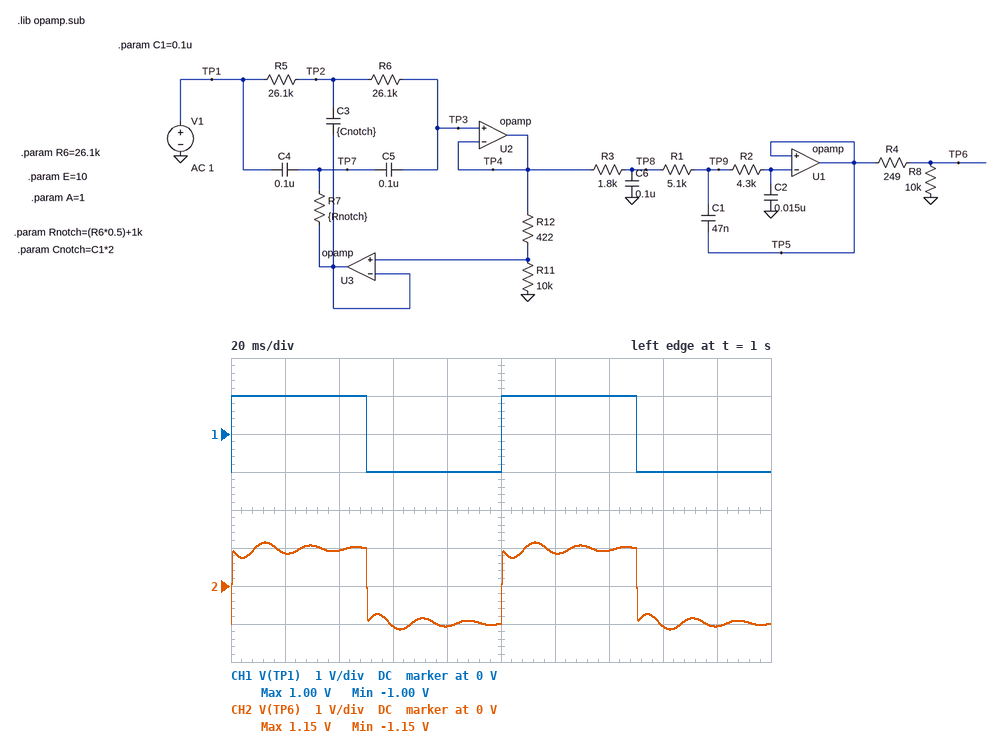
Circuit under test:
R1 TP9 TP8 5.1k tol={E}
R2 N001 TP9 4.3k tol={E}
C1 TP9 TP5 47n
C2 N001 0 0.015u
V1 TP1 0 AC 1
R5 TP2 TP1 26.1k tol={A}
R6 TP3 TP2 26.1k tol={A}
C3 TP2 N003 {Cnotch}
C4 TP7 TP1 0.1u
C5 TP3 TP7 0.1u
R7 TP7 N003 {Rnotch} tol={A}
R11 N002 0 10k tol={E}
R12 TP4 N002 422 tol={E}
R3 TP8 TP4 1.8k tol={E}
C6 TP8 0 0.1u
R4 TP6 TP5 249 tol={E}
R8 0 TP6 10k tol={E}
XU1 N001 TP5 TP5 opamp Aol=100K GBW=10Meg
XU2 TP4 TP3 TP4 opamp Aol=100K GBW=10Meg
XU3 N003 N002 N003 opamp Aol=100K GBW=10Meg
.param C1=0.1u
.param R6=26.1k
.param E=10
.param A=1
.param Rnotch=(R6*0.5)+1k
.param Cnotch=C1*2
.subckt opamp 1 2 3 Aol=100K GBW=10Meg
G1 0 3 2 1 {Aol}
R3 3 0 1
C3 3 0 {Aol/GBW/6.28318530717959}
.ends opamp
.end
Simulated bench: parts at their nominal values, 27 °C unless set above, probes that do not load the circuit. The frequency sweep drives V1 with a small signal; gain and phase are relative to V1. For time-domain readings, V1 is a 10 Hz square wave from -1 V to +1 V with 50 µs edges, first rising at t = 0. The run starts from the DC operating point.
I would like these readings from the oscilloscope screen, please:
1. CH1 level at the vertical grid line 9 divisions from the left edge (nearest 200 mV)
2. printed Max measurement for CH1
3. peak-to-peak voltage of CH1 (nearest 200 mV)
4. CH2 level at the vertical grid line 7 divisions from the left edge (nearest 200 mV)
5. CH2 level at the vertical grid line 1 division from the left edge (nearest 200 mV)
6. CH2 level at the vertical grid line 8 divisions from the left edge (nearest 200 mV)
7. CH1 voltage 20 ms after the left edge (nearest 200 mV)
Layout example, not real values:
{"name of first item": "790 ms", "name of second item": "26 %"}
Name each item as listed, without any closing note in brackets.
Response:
{"CH1 level at the vertical grid line 9 divisions from the left edge": "-1.0 V", "printed Max measurement for CH1": "1.00 V", "peak-to-peak voltage of CH1": "2.0 V", "CH2 level at the vertical grid line 7 divisions from the left edge": "1.0 V", "CH2 level at the vertical grid line 1 division from the left edge": "800 mV", "CH2 level at the vertical grid line 8 divisions from the left edge": "-1.0 V", "CH1 voltage 20 ms after the left edge": "1.0 V"}
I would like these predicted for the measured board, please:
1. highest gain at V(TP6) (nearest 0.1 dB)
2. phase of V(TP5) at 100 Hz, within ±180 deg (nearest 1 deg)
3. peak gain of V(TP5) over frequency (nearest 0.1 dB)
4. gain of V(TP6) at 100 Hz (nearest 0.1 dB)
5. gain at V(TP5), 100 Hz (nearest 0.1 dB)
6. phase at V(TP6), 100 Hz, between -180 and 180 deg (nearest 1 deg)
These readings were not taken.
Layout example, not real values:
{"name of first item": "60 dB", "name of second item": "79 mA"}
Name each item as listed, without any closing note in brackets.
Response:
{"highest gain at V(TP6)": "-0.2 dB", "phase of V(TP5) at 100 Hz, within ±180 deg": "-4 deg", "peak gain of V(TP5) over frequency": "0 dB", "gain of V(TP6) at 100 Hz": "-0.4 dB", "gain at V(TP5), 100 Hz": "-0.2 dB", "phase at V(TP6), 100 Hz, between -180 and 180 deg": "-4 deg"}
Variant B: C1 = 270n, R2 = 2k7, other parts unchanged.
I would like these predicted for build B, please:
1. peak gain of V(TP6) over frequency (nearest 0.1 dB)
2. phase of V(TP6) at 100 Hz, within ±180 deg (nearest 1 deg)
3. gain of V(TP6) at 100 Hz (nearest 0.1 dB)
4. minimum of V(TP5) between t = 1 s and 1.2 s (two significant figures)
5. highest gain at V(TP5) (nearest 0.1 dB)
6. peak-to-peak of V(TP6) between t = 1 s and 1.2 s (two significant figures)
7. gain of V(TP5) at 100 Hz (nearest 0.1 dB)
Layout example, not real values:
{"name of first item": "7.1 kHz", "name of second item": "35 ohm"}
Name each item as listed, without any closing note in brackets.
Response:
{"peak gain of V(TP6) over frequency": "2.8 dB", "phase of V(TP6) at 100 Hz, within ±180 deg": "-3 deg", "gain of V(TP6) at 100 Hz": "-0.2 dB", "minimum of V(TP5) between t = 1 s and 1.2 s": "-1.5 V", "highest gain at V(TP5)": "3.0 dB", "peak-to-peak of V(TP6) between t = 1 s and 1.2 s": "2.9 V", "gain of V(TP5) at 100 Hz": "0 dB"}
